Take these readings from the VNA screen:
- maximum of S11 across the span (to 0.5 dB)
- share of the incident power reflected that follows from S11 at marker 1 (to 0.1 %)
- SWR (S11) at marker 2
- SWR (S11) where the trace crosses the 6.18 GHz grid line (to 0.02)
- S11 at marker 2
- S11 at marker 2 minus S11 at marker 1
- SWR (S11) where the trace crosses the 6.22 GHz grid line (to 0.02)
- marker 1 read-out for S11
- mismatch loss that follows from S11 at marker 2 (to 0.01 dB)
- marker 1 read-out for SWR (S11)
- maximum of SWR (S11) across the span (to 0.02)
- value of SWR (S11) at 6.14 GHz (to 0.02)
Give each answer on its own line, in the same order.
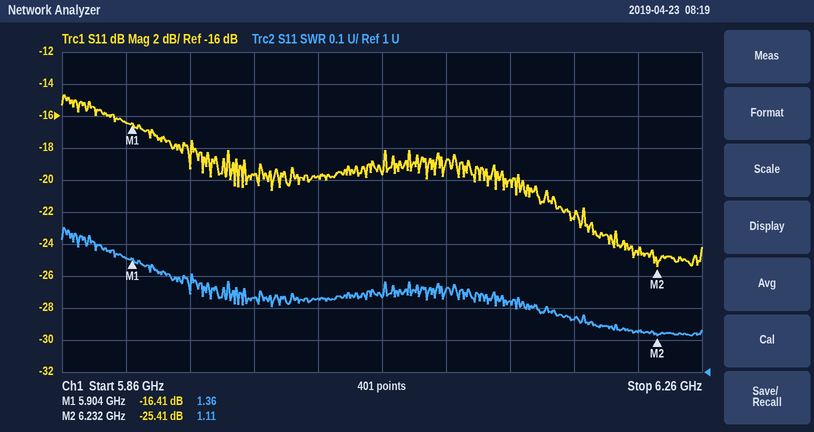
-14.5 dB
2.3 %
1.11
1.16
-25.41 dB
-9.00 dB
1.12
-16.41 dB
0.01 dB
1.36
1.46
1.22
